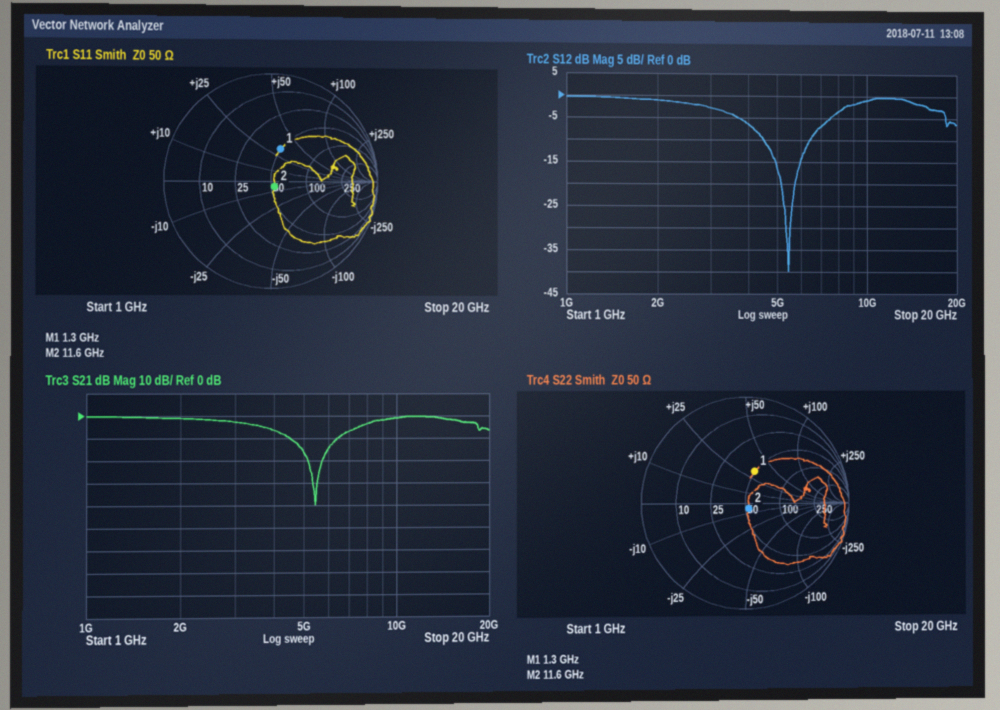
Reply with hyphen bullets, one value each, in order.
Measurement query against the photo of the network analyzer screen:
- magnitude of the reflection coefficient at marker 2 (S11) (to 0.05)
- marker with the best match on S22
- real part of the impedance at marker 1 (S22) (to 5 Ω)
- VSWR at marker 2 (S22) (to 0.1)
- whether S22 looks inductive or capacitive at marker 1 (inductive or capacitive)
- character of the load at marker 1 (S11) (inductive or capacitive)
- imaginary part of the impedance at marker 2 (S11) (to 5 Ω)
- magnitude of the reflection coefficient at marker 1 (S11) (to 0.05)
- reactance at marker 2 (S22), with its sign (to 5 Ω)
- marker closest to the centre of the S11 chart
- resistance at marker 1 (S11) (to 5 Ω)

- 0.05
- marker 2
- 50 Ω
- 1.1
- inductive
- inductive
- -5 Ω
- 0.30
- -5 Ω
- marker 2
- 50 Ω
